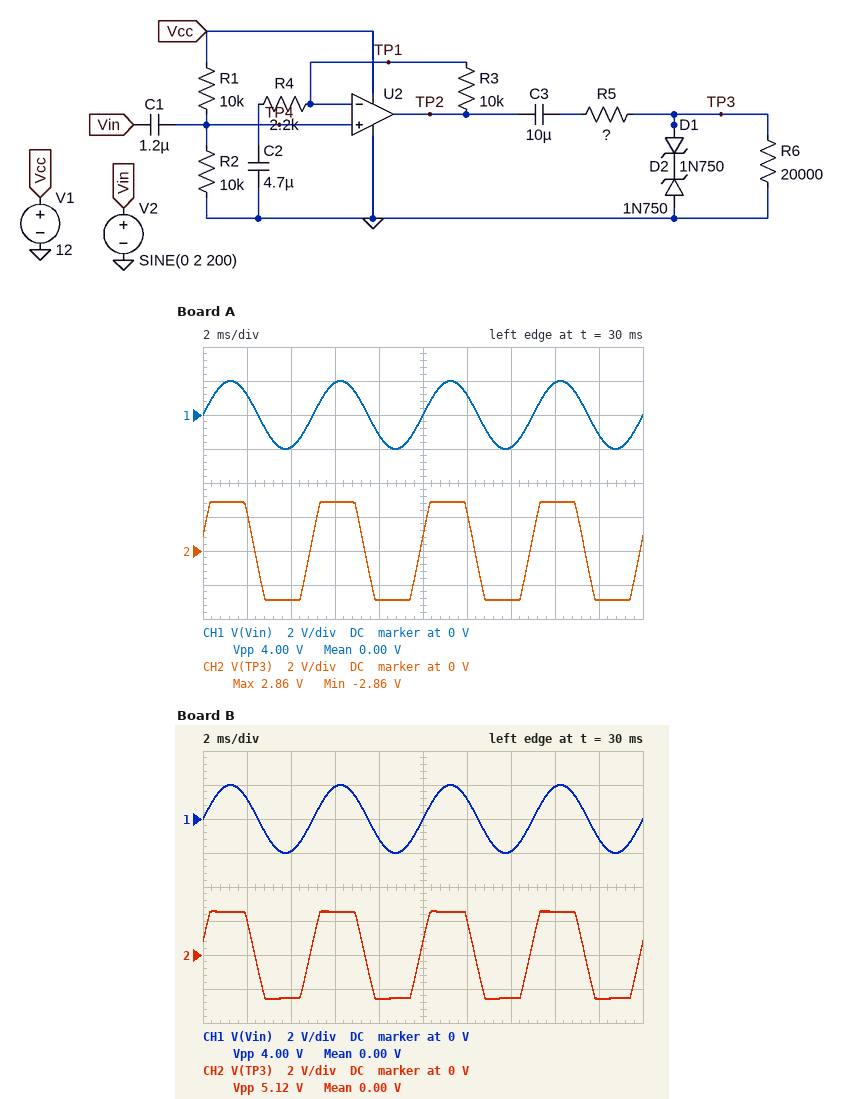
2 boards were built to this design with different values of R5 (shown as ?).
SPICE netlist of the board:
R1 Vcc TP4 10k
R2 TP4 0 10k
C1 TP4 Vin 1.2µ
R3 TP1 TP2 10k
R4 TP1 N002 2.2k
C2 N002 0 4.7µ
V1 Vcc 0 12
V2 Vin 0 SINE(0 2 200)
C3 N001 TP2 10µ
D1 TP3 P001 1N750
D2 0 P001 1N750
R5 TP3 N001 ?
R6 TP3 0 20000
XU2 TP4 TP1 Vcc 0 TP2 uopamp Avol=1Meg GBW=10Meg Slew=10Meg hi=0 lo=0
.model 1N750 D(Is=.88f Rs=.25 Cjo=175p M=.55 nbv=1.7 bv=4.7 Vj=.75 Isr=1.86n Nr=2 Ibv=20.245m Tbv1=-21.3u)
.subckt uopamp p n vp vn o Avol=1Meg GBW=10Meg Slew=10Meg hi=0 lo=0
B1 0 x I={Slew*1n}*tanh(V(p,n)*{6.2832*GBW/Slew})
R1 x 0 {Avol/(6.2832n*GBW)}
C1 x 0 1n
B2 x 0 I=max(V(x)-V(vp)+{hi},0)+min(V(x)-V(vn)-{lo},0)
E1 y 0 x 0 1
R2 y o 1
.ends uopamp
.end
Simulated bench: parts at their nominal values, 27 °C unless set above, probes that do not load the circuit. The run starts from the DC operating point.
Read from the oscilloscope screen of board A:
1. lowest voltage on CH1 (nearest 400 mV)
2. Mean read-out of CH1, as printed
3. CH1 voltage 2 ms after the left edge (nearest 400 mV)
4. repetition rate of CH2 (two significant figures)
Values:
-2.0 V
0.00 V
1.2 V
200 Hz
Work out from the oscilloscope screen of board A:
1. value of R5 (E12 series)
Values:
22 kΩ
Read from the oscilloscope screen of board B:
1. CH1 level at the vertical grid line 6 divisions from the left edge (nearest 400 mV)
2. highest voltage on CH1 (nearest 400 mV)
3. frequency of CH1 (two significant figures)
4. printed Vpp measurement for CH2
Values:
1.2 V
2.0 V
200 Hz
5.12 V
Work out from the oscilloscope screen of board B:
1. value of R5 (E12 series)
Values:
27 kΩ
